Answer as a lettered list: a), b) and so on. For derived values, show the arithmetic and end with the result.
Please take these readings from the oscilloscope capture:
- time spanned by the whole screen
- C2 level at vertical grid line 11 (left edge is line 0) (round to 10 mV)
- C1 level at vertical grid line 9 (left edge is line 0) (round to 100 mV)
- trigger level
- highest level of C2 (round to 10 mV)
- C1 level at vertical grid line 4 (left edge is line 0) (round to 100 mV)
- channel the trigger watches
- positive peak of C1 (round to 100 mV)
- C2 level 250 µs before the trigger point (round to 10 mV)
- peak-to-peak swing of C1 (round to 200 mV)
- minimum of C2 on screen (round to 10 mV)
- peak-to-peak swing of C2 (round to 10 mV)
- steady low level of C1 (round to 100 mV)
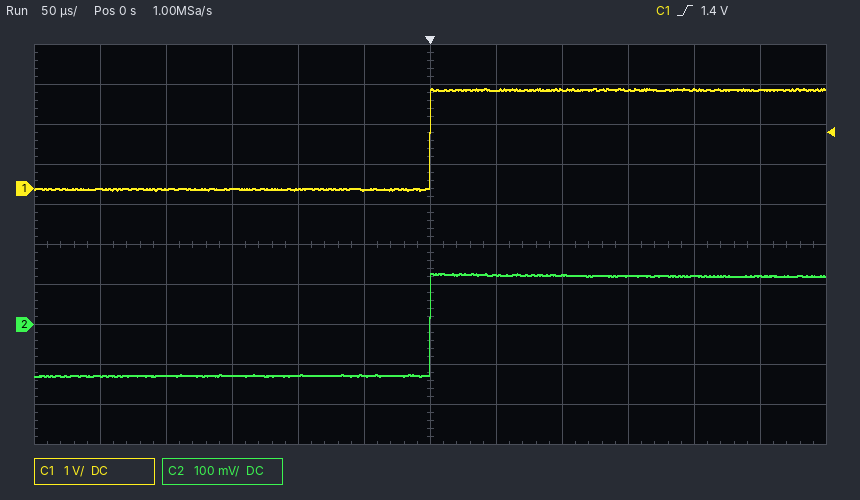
a) 600 µs
b) 120 mV
c) 2.5 V
d) 1.4 V
e) 130 mV
f) 0.0 V
g) C1
h) 2.5 V
i) -130 mV
j) 2.6 V
k) -130 mV
l) 130 mV − (-130 mV) = 260 mV
m) 0.0 V
